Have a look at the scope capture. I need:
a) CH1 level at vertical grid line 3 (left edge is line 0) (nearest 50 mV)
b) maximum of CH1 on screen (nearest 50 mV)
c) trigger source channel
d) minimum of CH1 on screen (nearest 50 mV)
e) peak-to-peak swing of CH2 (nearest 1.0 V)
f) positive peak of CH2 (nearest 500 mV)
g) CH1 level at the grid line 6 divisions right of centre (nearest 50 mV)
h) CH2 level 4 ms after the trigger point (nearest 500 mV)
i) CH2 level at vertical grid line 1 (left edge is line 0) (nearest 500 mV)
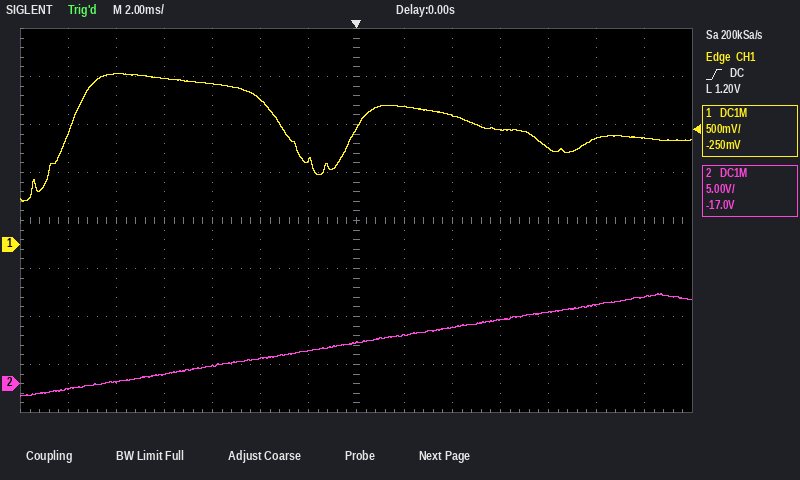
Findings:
1.75 V
1.80 V
CH1
450 mV
11.0 V
9.5 V
1.10 V
6.0 V
-500 mV
